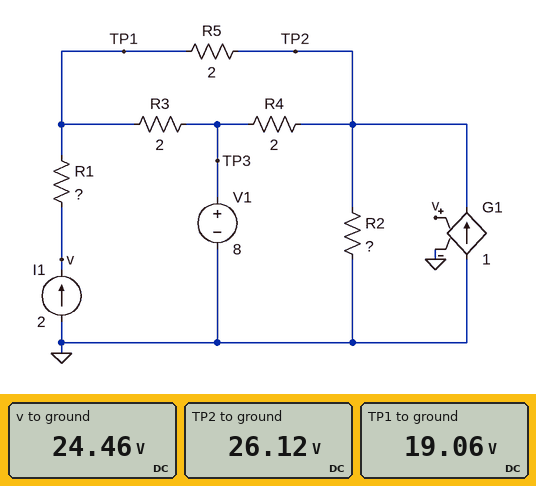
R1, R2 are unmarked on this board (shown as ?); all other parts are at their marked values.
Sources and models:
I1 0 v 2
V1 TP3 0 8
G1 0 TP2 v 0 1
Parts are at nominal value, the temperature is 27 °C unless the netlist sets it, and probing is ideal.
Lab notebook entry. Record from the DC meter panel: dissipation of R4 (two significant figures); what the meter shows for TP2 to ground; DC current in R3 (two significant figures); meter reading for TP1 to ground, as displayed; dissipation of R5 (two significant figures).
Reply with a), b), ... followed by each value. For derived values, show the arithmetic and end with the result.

a) (26.12 V - 8 V)^2 / 2 Ω = 160 W
b) 26.12 V
c) (19.06 V - 8 V) / 2 Ω = 5.5 A
d) 19.06 V
e) (26.12 V - 19.06 V)^2 / 2 Ω = 25 W
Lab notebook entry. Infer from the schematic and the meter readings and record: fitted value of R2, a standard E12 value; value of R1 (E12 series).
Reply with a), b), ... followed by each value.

a) 2.2 Ω
b) 2.7 Ω
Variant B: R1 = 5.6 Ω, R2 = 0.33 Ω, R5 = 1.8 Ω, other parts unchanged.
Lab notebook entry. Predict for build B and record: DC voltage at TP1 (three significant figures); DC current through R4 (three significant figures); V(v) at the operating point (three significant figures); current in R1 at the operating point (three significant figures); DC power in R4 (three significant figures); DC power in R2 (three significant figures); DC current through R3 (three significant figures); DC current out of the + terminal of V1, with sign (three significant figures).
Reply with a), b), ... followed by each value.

a) 9.56 V
b) 321 mA
c) 20.8 V
d) 2.00 A
e) 206 mW
f) 164 W
g) 779 mA
h) -458 mA
